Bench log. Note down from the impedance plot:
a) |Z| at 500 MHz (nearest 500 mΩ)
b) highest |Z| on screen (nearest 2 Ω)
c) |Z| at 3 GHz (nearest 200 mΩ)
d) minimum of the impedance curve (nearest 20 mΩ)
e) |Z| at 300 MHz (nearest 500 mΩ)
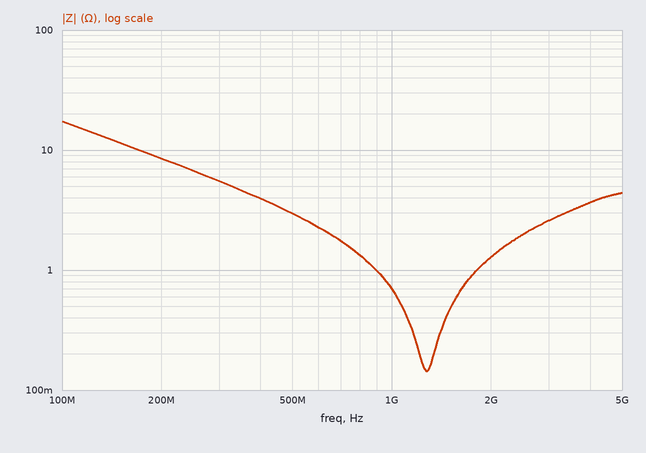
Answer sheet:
3.0 Ω
18 Ω
2.6 Ω
140 mΩ
5.5 Ω
